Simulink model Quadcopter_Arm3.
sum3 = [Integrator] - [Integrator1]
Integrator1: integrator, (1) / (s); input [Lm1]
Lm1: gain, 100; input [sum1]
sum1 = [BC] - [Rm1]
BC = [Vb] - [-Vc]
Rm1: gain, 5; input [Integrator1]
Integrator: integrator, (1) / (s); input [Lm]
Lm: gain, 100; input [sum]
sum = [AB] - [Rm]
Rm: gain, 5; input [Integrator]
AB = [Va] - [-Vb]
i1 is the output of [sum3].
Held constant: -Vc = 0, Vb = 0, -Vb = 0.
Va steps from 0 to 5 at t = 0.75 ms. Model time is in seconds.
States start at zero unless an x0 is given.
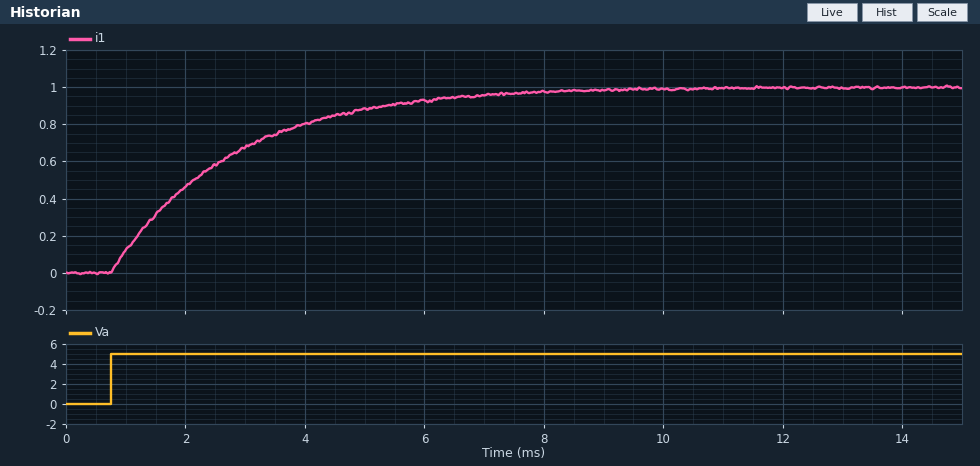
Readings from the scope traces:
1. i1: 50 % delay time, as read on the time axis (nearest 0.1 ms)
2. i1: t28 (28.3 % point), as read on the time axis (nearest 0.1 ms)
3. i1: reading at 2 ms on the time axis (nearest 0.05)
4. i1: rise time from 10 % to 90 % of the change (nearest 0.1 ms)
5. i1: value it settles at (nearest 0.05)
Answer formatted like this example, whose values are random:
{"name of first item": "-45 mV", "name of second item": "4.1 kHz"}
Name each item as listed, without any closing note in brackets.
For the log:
{"i1: 50 % delay time, as read on the time axis": "2.1 ms", "i1: t28 (28.3 % point), as read on the time axis": "1.4 ms", "i1: reading at 2 ms on the time axis": "0.45", "i1: rise time from 10 % to 90 % of the change": "4.4 ms", "i1: value it settles at": "1.00"}
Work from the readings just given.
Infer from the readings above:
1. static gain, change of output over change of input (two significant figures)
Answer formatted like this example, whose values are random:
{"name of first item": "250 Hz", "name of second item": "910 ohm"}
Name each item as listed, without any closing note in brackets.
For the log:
{"static gain, change of output over change of input": "0.20"}
